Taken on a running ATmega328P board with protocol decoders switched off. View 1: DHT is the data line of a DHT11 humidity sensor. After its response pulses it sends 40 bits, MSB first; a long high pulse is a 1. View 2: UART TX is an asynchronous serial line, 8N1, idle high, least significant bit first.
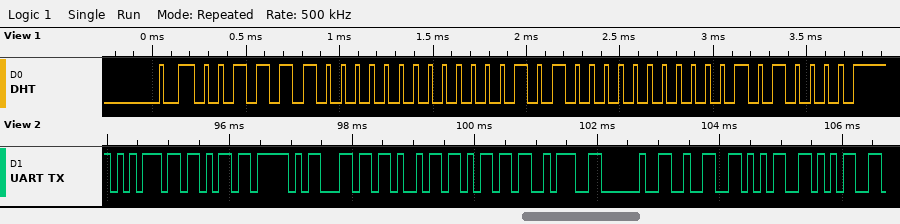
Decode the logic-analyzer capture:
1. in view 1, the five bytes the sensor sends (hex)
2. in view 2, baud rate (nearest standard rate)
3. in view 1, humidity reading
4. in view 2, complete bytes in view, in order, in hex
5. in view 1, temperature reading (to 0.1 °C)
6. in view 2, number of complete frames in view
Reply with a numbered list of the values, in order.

1. 3C 00 14 00 50
2. 9600 baud
3. 60 %
4. 75 6B 5F 6C 69 6D 3A 20 32 35 35
5. 20.0 °C
6. 11
